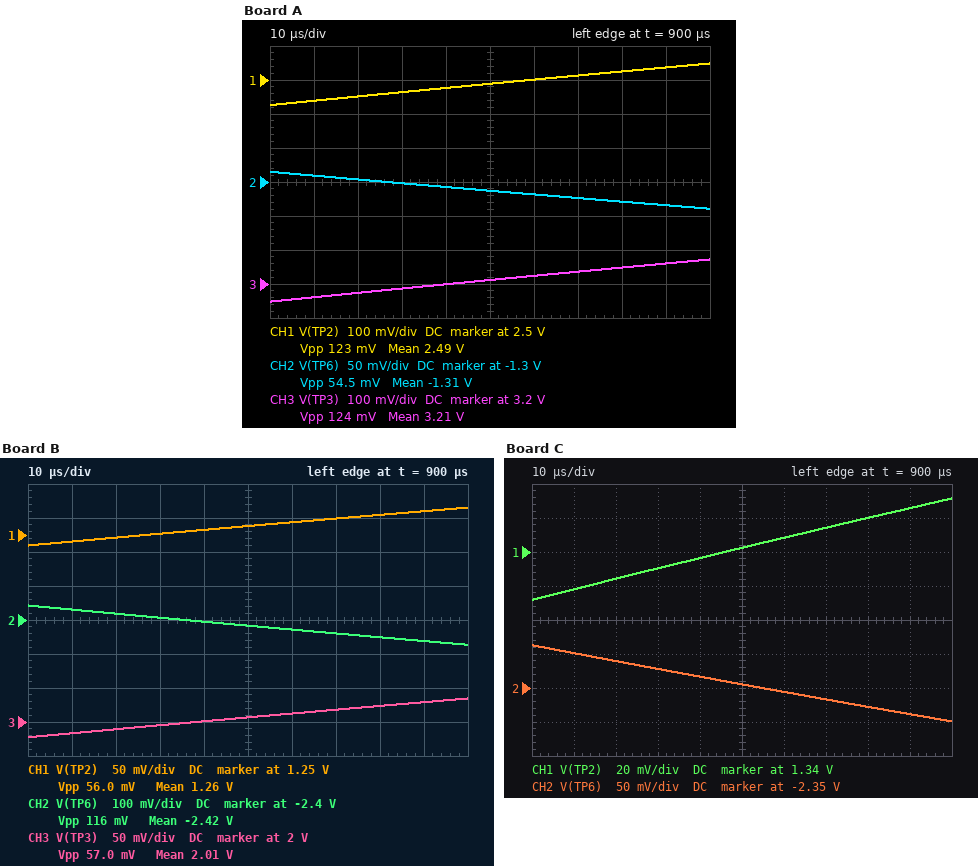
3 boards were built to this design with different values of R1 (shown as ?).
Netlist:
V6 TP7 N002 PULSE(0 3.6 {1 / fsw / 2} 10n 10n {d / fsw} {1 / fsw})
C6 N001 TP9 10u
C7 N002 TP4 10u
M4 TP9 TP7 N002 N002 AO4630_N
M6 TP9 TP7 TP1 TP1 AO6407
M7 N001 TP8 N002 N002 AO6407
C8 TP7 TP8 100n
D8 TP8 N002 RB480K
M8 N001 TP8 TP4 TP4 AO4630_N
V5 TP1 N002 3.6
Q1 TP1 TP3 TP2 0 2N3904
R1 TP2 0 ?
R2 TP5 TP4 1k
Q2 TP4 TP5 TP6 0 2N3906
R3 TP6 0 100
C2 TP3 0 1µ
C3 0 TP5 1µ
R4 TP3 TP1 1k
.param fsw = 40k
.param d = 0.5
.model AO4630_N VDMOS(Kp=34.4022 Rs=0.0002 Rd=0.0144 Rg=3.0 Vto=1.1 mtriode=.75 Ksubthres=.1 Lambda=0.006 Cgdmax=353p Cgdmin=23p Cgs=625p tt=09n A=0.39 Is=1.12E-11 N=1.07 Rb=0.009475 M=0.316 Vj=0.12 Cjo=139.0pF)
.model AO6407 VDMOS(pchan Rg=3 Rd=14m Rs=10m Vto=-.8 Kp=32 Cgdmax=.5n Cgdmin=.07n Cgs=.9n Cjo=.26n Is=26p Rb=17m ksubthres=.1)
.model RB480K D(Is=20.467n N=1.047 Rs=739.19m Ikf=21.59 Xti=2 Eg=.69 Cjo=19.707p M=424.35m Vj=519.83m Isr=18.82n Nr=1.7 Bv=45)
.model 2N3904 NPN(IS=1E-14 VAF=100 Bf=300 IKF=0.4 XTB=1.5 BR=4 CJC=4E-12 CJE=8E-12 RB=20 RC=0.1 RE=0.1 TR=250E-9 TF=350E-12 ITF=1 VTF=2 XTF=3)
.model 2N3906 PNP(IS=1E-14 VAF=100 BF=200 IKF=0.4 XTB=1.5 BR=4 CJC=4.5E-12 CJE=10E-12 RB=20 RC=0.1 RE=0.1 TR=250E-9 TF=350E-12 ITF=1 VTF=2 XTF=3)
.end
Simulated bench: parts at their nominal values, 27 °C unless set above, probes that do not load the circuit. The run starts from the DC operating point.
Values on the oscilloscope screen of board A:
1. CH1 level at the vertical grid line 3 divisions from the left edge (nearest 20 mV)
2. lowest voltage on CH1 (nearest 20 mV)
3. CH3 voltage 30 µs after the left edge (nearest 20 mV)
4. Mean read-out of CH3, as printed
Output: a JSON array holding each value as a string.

["2.46 V", "2.42 V", "3.18 V", "3.21 V"]
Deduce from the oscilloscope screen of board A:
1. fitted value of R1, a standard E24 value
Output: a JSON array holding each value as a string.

["200 Ω"]
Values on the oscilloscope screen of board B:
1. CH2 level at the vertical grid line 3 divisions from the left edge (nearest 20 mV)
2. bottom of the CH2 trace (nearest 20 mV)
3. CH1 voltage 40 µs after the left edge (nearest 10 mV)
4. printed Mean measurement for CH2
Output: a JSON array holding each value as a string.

["-2.40 V", "-2.48 V", "1.26 V", "-2.42 V"]
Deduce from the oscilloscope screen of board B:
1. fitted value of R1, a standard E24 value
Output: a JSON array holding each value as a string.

["51 Ω"]
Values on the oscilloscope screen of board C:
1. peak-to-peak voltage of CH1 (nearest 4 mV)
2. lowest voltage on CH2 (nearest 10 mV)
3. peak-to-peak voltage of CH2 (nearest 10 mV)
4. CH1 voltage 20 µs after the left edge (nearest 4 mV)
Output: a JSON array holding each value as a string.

["60 mV", "-2.40 V", "110 mV", "1.324 V"]
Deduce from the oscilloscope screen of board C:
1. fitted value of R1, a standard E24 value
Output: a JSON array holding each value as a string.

["56 Ω"]
